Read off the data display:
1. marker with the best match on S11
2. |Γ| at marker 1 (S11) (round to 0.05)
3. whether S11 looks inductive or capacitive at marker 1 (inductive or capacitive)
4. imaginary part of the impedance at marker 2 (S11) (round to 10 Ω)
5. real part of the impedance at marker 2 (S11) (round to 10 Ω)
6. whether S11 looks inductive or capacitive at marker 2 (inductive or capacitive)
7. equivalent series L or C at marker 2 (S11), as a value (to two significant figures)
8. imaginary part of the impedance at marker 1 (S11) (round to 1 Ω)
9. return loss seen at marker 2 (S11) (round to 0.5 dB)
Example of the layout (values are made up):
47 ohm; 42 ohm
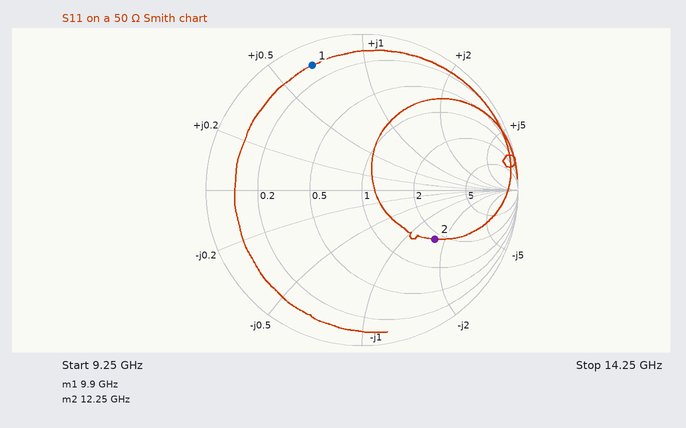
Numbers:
marker 2; 0.85; inductive; -80 Ω; 90 Ω; capacitive; 160 fF; +34 Ω; 5.0 dB
